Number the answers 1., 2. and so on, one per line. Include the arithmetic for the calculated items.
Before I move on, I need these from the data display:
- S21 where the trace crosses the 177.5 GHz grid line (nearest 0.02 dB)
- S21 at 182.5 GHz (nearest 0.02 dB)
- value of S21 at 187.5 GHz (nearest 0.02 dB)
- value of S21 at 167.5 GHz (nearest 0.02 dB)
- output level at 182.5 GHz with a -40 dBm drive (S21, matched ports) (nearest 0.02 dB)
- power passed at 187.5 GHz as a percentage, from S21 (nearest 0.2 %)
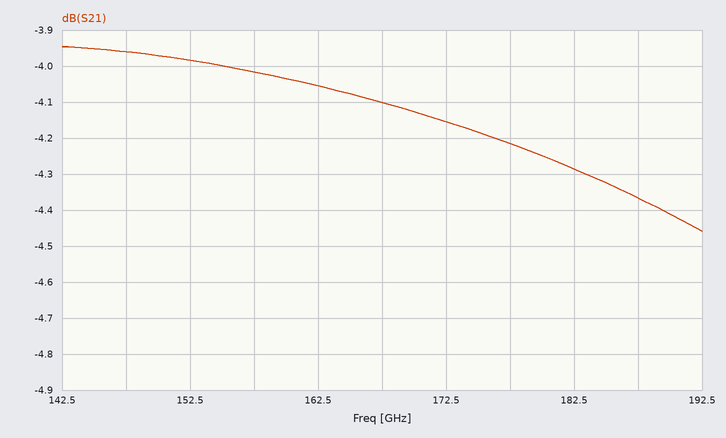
1. -4.22 dB
2. -4.28 dB
3. -4.36 dB
4. -4.10 dB
5. -40 dBm + (-4.28 dB) = -44.28 dBm
6. 10^(-4.36/10) ≈ 36.6 %
